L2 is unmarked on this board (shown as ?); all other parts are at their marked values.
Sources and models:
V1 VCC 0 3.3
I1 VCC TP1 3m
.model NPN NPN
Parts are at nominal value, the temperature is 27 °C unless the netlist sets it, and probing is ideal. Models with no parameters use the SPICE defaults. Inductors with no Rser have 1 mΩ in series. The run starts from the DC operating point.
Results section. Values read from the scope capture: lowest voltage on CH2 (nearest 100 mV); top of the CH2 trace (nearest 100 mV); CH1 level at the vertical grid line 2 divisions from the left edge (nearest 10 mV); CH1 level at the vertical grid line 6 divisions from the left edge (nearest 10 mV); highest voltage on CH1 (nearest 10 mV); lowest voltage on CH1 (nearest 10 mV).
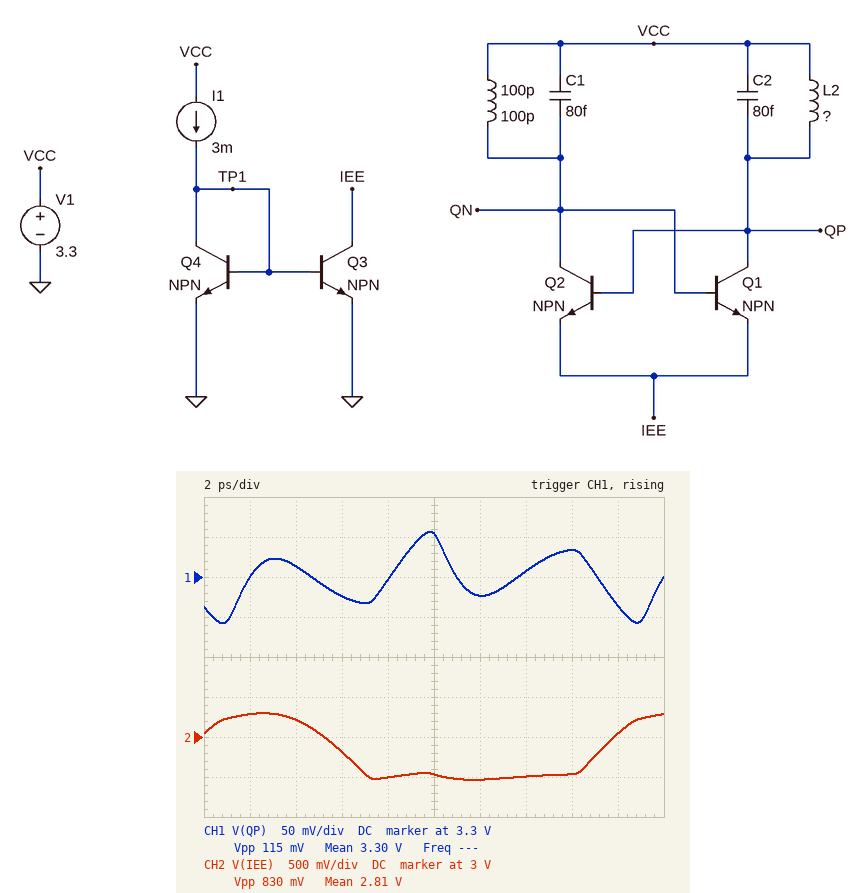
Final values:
2.5 V
3.3 V
3.31 V
3.28 V
3.36 V
3.24 V
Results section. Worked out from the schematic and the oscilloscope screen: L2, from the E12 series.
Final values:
33 pH
